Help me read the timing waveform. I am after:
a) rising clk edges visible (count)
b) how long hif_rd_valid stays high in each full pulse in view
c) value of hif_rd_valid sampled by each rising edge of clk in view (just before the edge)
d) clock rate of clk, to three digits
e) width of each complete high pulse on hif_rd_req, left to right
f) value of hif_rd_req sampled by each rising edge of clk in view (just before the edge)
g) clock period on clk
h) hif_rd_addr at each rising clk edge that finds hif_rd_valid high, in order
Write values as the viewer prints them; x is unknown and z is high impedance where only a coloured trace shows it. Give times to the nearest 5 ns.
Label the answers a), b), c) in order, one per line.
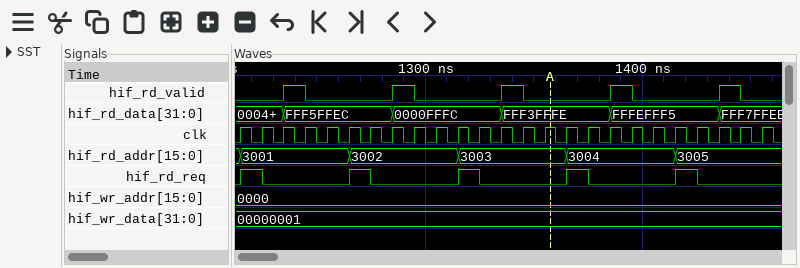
a) 25
b) 10 ns, 10 ns, 10 ns, 10 ns, 10 ns
c) 0 0 0 1 0 0 0 0 1 0 0 0 0 1 0 0 0 0 1 0 0 0 0 1 0
d) 100 MHz
e) 10 ns, 10 ns, 10 ns, 10 ns, 10 ns
f) 0 1 0 0 0 0 1 0 0 0 0 1 0 0 0 0 1 0 0 0 0 1 0 0 0
g) 10 ns
h) 3001, 3002, 3003, 3004, 3005
